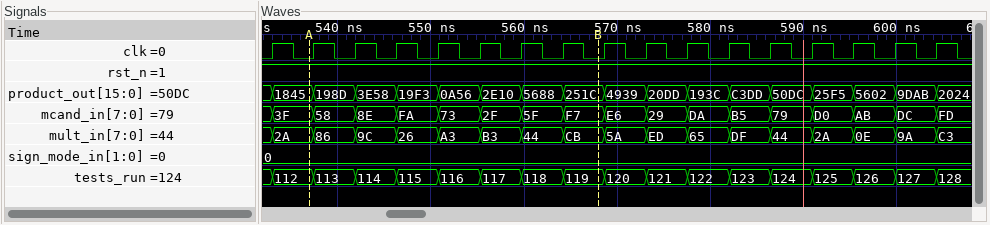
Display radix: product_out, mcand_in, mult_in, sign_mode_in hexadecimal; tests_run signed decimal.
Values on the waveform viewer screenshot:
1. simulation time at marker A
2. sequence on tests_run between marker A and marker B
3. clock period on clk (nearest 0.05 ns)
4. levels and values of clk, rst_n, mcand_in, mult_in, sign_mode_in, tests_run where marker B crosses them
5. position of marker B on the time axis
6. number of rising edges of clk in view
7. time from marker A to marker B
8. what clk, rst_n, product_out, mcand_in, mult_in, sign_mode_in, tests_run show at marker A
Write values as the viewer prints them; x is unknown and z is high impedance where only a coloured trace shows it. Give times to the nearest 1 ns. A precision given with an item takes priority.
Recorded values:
537 ns
112, 113, 114, 115, 116, 117, 118, 119
4.45 ns
clk=0, rst_n=1, mcand_in=F7, mult_in=CB, sign_mode_in=0, tests_run=119
568 ns
17
31 ns
clk=0, rst_n=1, product_out=1845, mcand_in=3F, mult_in=2A, sign_mode_in=0, tests_run=112
